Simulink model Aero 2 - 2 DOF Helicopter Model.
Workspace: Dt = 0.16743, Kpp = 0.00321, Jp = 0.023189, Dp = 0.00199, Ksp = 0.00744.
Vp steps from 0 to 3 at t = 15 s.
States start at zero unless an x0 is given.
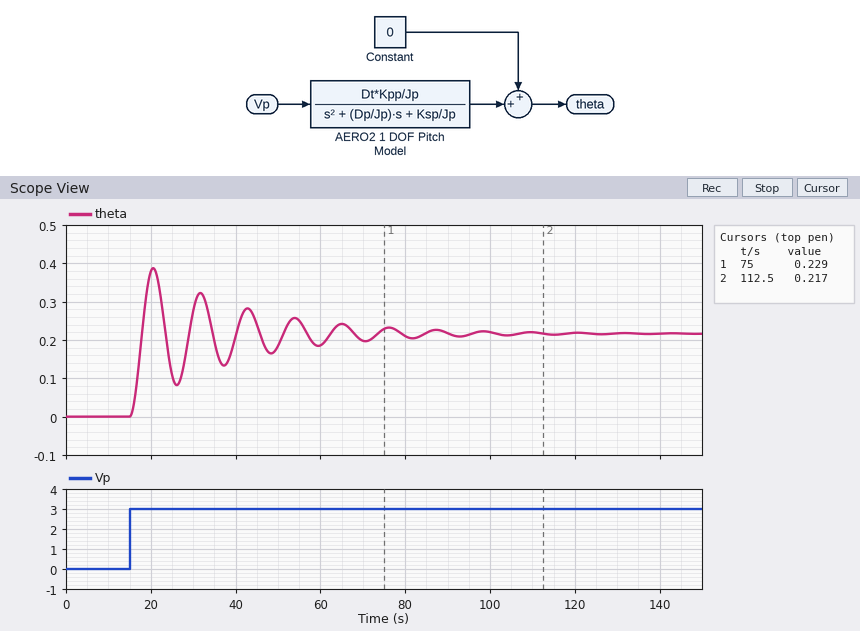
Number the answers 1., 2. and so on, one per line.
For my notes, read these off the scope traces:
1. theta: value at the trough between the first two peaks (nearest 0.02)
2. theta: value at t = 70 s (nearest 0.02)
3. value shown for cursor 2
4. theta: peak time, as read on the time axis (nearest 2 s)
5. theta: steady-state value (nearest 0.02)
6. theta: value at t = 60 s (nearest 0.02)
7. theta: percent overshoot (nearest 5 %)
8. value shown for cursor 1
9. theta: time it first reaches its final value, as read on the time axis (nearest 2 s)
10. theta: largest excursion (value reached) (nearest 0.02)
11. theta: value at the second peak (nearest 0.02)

1. 0.08
2. 0.20
3. 0.217
4. 20 s
5. 0.22
6. 0.18
7. 80 %
8. 0.229
9. 18 s
10. 0.38
11. 0.32
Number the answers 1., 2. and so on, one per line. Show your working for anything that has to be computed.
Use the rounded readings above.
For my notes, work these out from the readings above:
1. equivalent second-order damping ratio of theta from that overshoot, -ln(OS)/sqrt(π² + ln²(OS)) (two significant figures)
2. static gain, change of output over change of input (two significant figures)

1. ln(0.8) = -0.223; 0.223 / sqrt(9.870 + 0.050) = 0.071
2. (0.22 - 0) / (3 - 0) = 0.073
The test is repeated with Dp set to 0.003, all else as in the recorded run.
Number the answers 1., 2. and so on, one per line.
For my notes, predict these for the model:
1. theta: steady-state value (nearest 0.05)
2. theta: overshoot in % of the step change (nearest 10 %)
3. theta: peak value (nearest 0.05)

1. 0.20
2. 70 %
3. 0.35
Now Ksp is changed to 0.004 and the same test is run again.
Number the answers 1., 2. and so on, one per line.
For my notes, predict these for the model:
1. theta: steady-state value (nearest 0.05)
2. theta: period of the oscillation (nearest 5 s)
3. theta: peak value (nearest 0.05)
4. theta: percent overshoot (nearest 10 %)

1. 0.40
2. 15 s
3. 0.70
4. 70 %
